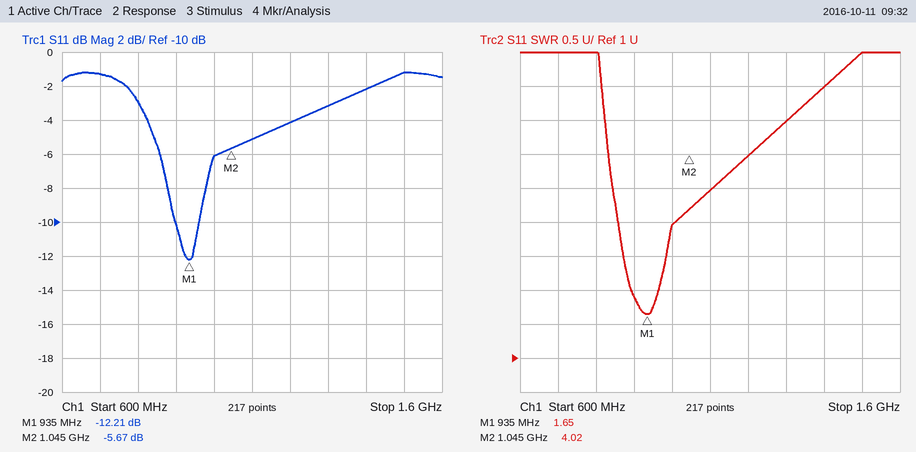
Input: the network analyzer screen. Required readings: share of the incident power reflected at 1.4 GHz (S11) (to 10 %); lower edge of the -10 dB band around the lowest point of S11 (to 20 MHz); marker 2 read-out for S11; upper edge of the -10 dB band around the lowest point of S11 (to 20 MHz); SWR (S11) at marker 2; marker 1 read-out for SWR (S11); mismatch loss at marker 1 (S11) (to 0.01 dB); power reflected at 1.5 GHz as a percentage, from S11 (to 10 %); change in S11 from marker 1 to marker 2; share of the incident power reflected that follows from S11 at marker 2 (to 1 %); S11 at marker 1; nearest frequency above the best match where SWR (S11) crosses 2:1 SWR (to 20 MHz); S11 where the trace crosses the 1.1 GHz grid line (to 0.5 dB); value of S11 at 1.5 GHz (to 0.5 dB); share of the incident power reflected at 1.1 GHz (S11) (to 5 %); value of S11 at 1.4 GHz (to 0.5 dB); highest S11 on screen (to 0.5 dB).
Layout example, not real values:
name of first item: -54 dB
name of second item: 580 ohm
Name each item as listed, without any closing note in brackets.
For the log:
share of the incident power reflected at 1.4 GHz (S11): 60 %
lower edge of the -10 dB band around the lowest point of S11: 900 MHz
marker 2 read-out for S11: -5.67 dB
upper edge of the -10 dB band around the lowest point of S11: 960 MHz
SWR (S11) at marker 2: 4.02
marker 1 read-out for SWR: 1.65
mismatch loss at marker 1 (S11): 0.27 dB
power reflected at 1.5 GHz as a percentage, from S11: 80 %
change in S11 from marker 1 to marker 2: 6.54 dB
share of the incident power reflected that follows from S11 at marker 2: 27 %
S11 at marker 1: -12.21 dB
nearest frequency above the best match where SWR (S11) crosses 2:1 SWR: 960 MHz
S11 where the trace crosses the 1.1 GHz grid line: -5.0 dB
value of S11 at 1.5 GHz: -1.0 dB
share of the incident power reflected at 1.1 GHz (S11): 30 %
value of S11 at 1.4 GHz: -2.0 dB
highest S11 on screen: -1.0 dB
